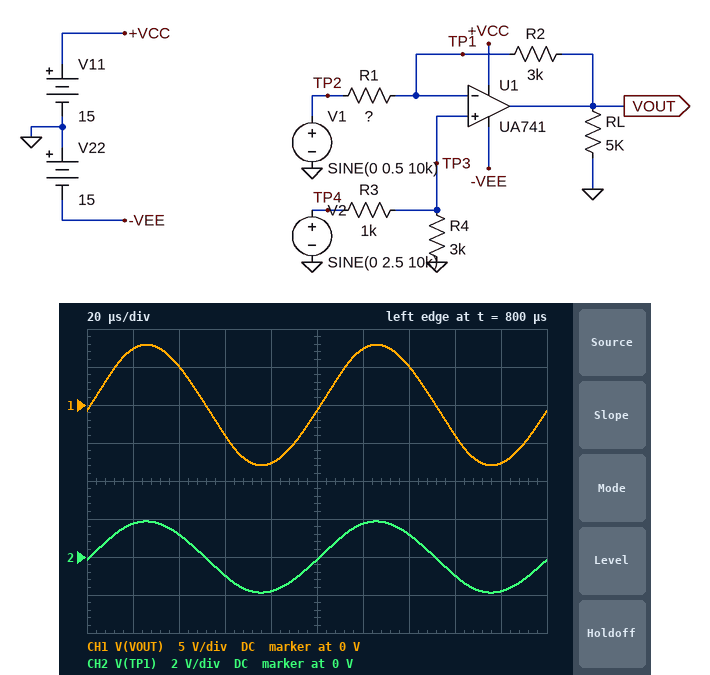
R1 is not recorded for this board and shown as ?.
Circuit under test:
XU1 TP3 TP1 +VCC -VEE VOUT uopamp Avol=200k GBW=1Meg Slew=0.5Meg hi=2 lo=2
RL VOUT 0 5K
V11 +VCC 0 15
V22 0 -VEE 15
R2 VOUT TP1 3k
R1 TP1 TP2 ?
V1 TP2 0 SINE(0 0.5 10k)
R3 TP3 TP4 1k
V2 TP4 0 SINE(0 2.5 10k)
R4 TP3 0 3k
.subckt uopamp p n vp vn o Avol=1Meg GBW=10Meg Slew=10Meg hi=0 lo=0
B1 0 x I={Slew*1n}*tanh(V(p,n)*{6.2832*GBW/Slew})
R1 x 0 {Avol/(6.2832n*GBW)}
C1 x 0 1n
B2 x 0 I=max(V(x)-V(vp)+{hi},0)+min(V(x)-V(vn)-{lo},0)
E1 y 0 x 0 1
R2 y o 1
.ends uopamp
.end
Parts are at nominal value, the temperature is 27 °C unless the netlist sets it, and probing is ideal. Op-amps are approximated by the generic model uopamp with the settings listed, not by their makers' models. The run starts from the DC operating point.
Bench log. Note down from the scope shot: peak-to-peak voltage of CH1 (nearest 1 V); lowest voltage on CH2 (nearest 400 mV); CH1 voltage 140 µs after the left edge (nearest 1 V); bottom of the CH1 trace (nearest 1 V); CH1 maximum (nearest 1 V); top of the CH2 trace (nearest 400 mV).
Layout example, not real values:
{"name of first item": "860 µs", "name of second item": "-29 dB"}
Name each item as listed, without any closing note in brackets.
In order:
{"peak-to-peak voltage of CH1": "16 V", "lowest voltage on CH2": "-2.0 V", "CH1 voltage 140 µs after the left edge": "5 V", "bottom of the CH1 trace": "-8 V", "CH1 maximum": "8 V", "top of the CH2 trace": "2.0 V"}
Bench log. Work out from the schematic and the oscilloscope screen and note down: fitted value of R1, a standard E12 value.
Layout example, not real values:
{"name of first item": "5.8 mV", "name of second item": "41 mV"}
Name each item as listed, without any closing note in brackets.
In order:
{"fitted value of R1, a standard E12 value": "680 Ω"}
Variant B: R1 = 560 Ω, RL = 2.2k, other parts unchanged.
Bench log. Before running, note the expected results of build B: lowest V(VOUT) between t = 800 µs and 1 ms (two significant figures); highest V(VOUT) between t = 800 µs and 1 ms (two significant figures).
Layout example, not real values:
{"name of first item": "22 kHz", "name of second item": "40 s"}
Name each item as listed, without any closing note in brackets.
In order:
{"lowest V(VOUT) between t = 800 µs and 1 ms": "-9.2 V", "highest V(VOUT) between t = 800 µs and 1 ms": "9.2 V"}
